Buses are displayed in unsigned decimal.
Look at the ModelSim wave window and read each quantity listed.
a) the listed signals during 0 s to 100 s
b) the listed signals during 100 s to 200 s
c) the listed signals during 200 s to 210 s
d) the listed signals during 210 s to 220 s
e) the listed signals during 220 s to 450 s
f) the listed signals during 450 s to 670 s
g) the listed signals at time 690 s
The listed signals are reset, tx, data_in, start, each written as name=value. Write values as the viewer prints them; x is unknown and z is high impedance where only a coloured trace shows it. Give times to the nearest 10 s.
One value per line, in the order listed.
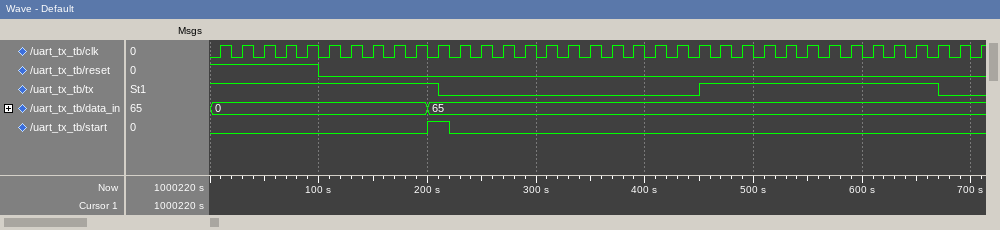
reset=1, tx=1, data_in=0, start=0
reset=0, tx=1, data_in=0, start=0
reset=0, tx=1, data_in=65, start=1
reset=0, tx=0, data_in=65, start=1
reset=0, tx=0, data_in=65, start=0
reset=0, tx=1, data_in=65, start=0
reset=0, tx=0, data_in=65, start=0
